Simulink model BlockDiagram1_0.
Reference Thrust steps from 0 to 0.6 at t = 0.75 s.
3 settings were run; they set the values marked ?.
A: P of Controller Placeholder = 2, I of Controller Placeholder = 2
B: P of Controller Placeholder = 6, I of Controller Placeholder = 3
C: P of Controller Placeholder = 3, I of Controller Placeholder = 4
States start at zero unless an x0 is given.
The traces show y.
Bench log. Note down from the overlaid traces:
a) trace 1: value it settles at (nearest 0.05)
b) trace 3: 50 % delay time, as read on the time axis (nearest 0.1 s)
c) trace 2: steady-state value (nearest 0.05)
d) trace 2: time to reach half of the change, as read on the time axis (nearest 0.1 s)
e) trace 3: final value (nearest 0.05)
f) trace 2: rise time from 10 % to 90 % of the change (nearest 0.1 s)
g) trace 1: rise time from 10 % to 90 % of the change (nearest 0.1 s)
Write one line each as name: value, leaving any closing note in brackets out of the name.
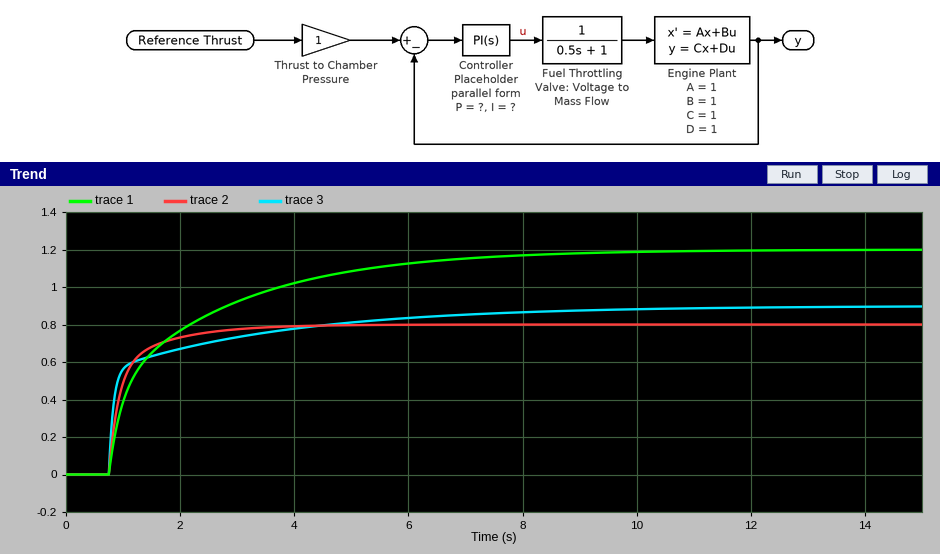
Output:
trace 1: value it settles at: 1.20
trace 3: 50 % delay time, as read on the time axis: 0.9 s
trace 2: steady-state value: 0.80
trace 2: time to reach half of the change, as read on the time axis: 0.9 s
trace 3: final value: 0.90
trace 2: rise time from 10 % to 90 % of the change: 1.1 s
trace 1: rise time from 10 % to 90 % of the change: 4.1 s
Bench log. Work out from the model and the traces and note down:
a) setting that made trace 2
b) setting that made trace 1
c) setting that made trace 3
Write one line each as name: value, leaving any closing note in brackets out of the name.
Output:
setting that made trace 2: C
setting that made trace 1: A
setting that made trace 3: B
